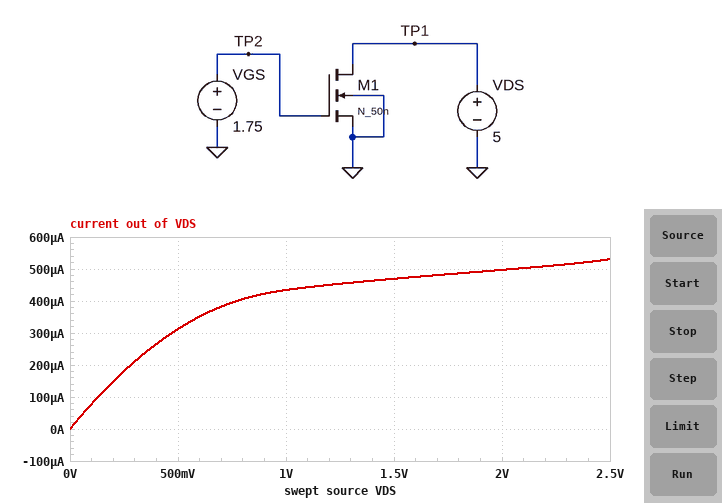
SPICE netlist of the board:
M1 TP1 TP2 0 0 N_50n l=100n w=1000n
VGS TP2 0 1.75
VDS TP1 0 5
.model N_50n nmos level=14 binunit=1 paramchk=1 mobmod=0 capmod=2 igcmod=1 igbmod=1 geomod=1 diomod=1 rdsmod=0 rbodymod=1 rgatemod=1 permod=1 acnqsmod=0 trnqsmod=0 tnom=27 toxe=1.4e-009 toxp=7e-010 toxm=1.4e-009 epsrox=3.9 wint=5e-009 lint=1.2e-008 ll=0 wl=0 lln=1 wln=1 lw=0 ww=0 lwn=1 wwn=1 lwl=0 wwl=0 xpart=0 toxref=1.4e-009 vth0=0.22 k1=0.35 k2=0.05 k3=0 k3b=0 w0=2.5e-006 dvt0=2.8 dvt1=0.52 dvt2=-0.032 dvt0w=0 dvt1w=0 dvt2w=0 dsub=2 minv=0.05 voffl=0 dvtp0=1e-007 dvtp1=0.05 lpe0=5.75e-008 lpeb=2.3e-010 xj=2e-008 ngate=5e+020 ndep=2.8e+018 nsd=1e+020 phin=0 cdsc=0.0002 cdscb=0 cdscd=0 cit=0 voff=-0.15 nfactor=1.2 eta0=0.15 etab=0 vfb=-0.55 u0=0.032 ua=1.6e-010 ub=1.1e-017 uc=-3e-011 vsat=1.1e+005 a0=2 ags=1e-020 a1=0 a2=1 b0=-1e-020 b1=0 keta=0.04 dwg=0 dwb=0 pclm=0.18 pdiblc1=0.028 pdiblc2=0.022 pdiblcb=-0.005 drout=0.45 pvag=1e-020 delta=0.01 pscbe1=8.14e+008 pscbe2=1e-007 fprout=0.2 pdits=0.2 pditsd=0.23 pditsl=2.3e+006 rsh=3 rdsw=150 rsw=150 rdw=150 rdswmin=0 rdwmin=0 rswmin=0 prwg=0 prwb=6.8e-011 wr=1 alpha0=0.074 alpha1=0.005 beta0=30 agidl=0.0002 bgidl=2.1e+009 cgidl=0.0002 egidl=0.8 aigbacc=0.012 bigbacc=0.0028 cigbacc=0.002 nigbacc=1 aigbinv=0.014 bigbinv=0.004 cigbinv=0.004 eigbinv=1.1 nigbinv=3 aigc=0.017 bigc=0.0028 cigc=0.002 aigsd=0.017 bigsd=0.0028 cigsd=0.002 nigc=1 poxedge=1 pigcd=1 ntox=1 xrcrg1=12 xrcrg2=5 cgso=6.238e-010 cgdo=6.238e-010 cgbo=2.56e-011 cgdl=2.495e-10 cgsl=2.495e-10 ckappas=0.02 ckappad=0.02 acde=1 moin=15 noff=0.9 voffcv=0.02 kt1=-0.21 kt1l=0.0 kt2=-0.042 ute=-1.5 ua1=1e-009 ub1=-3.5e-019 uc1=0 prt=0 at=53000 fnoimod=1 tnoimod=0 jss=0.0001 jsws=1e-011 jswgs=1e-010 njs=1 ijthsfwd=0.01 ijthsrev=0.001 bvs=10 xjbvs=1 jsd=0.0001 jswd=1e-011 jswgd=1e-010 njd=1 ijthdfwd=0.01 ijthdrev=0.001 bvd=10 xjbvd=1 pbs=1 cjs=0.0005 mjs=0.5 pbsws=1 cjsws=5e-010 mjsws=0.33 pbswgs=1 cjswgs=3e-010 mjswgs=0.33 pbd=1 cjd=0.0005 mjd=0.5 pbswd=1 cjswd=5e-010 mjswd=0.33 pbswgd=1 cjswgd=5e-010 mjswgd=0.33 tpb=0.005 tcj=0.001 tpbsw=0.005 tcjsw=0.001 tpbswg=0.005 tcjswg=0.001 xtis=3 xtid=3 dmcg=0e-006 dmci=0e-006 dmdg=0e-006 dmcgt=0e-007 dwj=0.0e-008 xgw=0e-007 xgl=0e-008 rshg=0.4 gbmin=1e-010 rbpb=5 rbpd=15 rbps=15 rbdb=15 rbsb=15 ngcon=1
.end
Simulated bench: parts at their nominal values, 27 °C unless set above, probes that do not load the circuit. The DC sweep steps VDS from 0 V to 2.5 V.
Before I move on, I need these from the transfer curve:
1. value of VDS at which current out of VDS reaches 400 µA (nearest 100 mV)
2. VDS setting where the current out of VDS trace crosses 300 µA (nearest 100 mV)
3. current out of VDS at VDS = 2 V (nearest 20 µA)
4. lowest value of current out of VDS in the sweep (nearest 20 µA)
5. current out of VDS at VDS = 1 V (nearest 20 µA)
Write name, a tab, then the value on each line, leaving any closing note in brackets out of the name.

value of VDS at which current out of VDS reaches 400 µA	800 mV
VDS setting where the current out of VDS trace crosses 300 µA	500 mV
current out of VDS at VDS = 2 V	500 µA
lowest value of current out of VDS in the sweep	0 A
current out of VDS at VDS = 1 V	440 µA
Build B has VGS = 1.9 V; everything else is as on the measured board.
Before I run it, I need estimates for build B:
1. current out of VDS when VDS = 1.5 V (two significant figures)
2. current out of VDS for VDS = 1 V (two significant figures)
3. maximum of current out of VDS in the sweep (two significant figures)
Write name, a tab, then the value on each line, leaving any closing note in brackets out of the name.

current out of VDS when VDS = 1.5 V	500 µA
current out of VDS for VDS = 1 V	460 µA
maximum of current out of VDS in the sweep	560 µA
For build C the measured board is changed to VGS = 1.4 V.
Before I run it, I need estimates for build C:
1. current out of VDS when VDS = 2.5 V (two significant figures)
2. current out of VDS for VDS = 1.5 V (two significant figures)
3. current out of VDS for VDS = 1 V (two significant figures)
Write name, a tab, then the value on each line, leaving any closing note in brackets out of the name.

current out of VDS when VDS = 2.5 V	470 µA
current out of VDS for VDS = 1.5 V	380 µA
current out of VDS for VDS = 1 V	350 µA
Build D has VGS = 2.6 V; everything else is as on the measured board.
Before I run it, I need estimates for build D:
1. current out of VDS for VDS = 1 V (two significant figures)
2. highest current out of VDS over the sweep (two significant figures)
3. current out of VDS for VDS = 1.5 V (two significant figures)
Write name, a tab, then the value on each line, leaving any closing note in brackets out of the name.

current out of VDS for VDS = 1 V	510 µA
highest current out of VDS over the sweep	670 µA
current out of VDS for VDS = 1.5 V	600 µA
